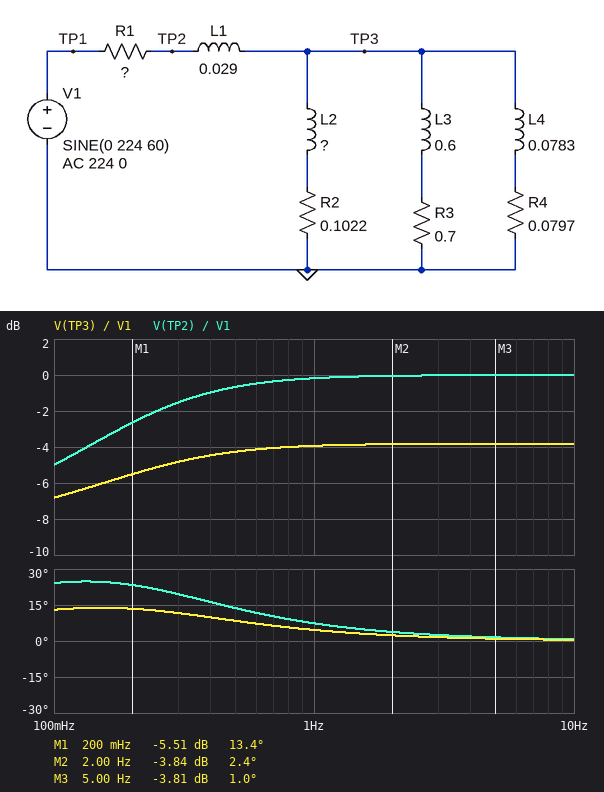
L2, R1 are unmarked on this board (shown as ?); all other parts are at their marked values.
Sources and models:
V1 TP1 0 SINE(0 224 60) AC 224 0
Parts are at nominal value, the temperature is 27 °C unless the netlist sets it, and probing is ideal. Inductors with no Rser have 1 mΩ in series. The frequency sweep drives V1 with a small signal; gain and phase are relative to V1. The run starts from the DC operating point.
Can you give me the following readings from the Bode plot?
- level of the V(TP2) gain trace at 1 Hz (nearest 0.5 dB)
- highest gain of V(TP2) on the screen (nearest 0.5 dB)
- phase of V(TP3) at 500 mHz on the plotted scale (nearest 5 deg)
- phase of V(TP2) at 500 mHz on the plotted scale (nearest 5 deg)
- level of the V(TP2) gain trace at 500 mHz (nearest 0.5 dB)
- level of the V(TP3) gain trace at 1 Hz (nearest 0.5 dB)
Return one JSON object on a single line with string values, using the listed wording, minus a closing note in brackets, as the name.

{"level of the V(TP2) gain trace at 1 Hz": "0 dB", "highest gain of V(TP2) on the screen": "0 dB", "phase of V(TP3) at 500 mHz on the plotted scale": "10 deg", "phase of V(TP2) at 500 mHz on the plotted scale": "15 deg", "level of the V(TP2) gain trace at 500 mHz": "-0.5 dB", "level of the V(TP3) gain trace at 1 Hz": "-4.0 dB"}
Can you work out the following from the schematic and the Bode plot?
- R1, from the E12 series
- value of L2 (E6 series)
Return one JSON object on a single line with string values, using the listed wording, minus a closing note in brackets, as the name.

{"R1, from the E12 series": "0.068 Ω", "value of L2": "220 mH"}
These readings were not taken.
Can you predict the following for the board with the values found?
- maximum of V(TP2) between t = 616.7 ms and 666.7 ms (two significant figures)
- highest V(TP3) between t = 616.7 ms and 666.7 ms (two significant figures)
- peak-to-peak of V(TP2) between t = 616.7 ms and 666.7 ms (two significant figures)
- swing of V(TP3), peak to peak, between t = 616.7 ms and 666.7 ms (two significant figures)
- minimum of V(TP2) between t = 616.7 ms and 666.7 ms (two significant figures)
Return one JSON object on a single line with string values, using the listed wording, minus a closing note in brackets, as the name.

{"maximum of V(TP2) between t = 616.7 ms and 666.7 ms": "220 V", "highest V(TP3) between t = 616.7 ms and 666.7 ms": "140 V", "peak-to-peak of V(TP2) between t = 616.7 ms and 666.7 ms": "450 V", "swing of V(TP3), peak to peak, between t = 616.7 ms and 666.7 ms": "290 V", "minimum of V(TP2) between t = 616.7 ms and 666.7 ms": "-220 V"}
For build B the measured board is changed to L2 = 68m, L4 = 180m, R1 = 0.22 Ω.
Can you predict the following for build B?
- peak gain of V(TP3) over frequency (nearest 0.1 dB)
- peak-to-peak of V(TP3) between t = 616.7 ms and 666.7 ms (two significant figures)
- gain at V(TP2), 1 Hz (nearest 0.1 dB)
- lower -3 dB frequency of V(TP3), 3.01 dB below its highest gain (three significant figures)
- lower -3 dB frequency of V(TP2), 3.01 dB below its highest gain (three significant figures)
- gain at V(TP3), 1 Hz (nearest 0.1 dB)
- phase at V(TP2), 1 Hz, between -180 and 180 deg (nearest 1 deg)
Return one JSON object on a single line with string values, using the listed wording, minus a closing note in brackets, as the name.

{"peak gain of V(TP3) over frequency": "-4.3 dB", "peak-to-peak of V(TP3) between t = 616.7 ms and 666.7 ms": "270 V", "gain at V(TP2), 1 Hz": "-1.2 dB", "lower -3 dB frequency of V(TP3), 3.01 dB below its highest gain": "509 mHz", "lower -3 dB frequency of V(TP2), 3.01 dB below its highest gain": "559 mHz", "gain at V(TP3), 1 Hz": "-5.4 dB", "phase at V(TP2), 1 Hz, between -180 and 180 deg": "24 deg"}
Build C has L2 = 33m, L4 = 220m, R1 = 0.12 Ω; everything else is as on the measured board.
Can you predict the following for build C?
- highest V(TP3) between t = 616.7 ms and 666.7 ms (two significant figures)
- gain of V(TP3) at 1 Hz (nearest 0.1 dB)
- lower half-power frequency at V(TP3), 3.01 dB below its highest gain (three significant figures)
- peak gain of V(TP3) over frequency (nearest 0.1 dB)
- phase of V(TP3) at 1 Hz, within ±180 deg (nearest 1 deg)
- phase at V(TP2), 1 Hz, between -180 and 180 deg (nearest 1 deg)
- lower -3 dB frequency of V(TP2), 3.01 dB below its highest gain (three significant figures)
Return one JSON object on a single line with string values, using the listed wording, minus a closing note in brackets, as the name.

{"highest V(TP3) between t = 616.7 ms and 666.7 ms": "110 V", "gain of V(TP3) at 1 Hz": "-6.6 dB", "lower half-power frequency at V(TP3), 3.01 dB below its highest gain": "94.0 mHz", "peak gain of V(TP3) over frequency": "-6.3 dB", "phase of V(TP3) at 1 Hz, within ±180 deg": "6 deg", "phase at V(TP2), 1 Hz, between -180 and 180 deg": "17 deg", "lower -3 dB frequency of V(TP2), 3.01 dB below its highest gain": "436 mHz"}
